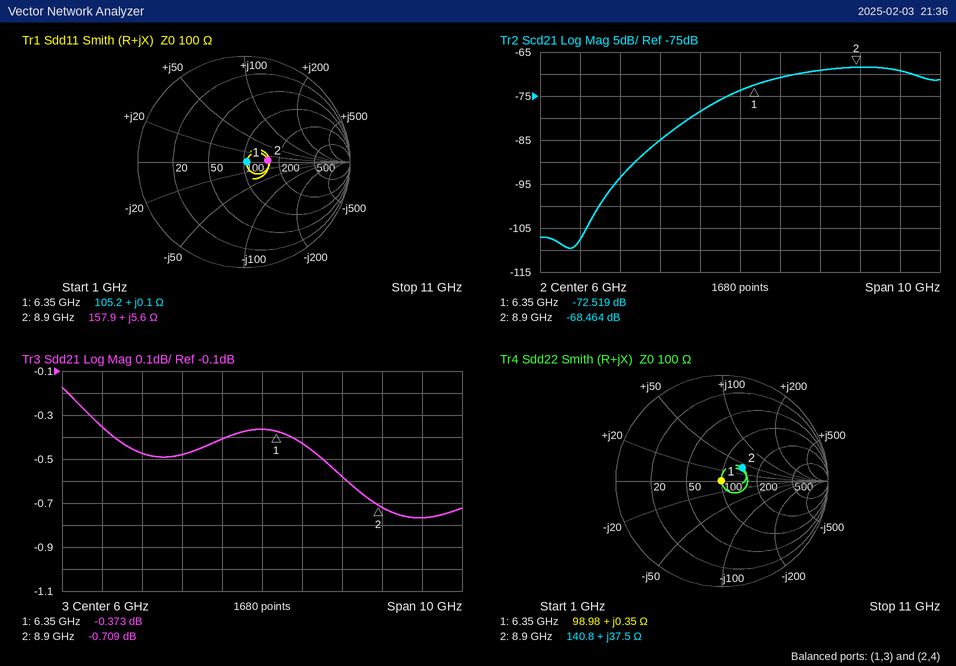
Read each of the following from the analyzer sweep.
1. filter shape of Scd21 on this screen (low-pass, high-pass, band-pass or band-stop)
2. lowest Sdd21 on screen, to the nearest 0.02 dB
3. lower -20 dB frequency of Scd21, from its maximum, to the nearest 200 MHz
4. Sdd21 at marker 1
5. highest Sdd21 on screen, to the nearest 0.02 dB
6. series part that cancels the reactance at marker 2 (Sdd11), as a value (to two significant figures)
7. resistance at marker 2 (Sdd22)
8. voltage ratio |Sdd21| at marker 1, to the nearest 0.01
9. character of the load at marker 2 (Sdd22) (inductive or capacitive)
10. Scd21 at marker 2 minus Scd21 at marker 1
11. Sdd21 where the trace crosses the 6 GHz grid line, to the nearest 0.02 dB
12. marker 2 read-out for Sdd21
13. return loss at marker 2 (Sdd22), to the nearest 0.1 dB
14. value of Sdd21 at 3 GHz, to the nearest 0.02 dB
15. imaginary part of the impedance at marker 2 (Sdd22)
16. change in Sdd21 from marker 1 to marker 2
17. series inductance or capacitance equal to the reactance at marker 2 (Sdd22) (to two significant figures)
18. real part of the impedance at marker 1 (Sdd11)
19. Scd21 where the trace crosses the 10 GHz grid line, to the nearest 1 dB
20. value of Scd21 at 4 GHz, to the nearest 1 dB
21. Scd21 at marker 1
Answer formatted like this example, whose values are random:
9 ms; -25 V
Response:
high-pass; -0.76 dB; 3.6 GHz; -0.373 dB; -0.18 dB; 3.2 pF; 140.8 Ω; 0.96; inductive; 4.055 dB; -0.36 dB; -0.709 dB; 12.9 dB; -0.48 dB; +37.5 Ω; -0.336 dB; 670 pH; 105.2 Ω; -69 dB; -85 dB; -72.519 dB
